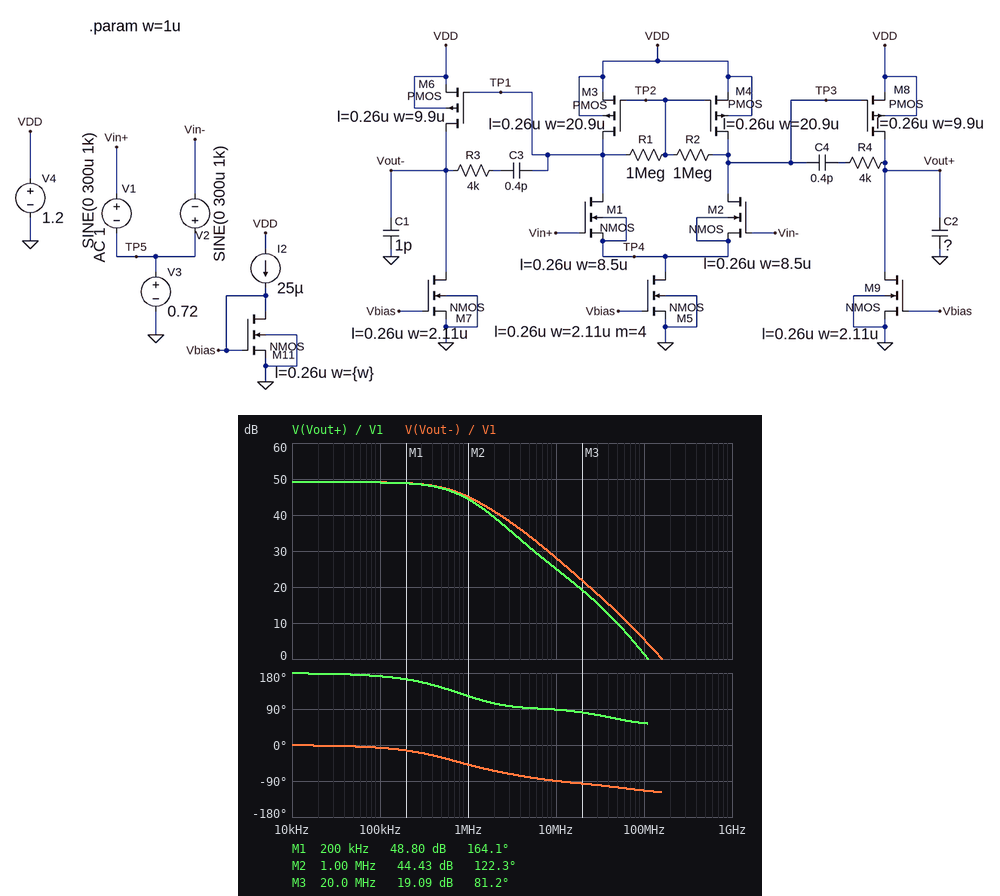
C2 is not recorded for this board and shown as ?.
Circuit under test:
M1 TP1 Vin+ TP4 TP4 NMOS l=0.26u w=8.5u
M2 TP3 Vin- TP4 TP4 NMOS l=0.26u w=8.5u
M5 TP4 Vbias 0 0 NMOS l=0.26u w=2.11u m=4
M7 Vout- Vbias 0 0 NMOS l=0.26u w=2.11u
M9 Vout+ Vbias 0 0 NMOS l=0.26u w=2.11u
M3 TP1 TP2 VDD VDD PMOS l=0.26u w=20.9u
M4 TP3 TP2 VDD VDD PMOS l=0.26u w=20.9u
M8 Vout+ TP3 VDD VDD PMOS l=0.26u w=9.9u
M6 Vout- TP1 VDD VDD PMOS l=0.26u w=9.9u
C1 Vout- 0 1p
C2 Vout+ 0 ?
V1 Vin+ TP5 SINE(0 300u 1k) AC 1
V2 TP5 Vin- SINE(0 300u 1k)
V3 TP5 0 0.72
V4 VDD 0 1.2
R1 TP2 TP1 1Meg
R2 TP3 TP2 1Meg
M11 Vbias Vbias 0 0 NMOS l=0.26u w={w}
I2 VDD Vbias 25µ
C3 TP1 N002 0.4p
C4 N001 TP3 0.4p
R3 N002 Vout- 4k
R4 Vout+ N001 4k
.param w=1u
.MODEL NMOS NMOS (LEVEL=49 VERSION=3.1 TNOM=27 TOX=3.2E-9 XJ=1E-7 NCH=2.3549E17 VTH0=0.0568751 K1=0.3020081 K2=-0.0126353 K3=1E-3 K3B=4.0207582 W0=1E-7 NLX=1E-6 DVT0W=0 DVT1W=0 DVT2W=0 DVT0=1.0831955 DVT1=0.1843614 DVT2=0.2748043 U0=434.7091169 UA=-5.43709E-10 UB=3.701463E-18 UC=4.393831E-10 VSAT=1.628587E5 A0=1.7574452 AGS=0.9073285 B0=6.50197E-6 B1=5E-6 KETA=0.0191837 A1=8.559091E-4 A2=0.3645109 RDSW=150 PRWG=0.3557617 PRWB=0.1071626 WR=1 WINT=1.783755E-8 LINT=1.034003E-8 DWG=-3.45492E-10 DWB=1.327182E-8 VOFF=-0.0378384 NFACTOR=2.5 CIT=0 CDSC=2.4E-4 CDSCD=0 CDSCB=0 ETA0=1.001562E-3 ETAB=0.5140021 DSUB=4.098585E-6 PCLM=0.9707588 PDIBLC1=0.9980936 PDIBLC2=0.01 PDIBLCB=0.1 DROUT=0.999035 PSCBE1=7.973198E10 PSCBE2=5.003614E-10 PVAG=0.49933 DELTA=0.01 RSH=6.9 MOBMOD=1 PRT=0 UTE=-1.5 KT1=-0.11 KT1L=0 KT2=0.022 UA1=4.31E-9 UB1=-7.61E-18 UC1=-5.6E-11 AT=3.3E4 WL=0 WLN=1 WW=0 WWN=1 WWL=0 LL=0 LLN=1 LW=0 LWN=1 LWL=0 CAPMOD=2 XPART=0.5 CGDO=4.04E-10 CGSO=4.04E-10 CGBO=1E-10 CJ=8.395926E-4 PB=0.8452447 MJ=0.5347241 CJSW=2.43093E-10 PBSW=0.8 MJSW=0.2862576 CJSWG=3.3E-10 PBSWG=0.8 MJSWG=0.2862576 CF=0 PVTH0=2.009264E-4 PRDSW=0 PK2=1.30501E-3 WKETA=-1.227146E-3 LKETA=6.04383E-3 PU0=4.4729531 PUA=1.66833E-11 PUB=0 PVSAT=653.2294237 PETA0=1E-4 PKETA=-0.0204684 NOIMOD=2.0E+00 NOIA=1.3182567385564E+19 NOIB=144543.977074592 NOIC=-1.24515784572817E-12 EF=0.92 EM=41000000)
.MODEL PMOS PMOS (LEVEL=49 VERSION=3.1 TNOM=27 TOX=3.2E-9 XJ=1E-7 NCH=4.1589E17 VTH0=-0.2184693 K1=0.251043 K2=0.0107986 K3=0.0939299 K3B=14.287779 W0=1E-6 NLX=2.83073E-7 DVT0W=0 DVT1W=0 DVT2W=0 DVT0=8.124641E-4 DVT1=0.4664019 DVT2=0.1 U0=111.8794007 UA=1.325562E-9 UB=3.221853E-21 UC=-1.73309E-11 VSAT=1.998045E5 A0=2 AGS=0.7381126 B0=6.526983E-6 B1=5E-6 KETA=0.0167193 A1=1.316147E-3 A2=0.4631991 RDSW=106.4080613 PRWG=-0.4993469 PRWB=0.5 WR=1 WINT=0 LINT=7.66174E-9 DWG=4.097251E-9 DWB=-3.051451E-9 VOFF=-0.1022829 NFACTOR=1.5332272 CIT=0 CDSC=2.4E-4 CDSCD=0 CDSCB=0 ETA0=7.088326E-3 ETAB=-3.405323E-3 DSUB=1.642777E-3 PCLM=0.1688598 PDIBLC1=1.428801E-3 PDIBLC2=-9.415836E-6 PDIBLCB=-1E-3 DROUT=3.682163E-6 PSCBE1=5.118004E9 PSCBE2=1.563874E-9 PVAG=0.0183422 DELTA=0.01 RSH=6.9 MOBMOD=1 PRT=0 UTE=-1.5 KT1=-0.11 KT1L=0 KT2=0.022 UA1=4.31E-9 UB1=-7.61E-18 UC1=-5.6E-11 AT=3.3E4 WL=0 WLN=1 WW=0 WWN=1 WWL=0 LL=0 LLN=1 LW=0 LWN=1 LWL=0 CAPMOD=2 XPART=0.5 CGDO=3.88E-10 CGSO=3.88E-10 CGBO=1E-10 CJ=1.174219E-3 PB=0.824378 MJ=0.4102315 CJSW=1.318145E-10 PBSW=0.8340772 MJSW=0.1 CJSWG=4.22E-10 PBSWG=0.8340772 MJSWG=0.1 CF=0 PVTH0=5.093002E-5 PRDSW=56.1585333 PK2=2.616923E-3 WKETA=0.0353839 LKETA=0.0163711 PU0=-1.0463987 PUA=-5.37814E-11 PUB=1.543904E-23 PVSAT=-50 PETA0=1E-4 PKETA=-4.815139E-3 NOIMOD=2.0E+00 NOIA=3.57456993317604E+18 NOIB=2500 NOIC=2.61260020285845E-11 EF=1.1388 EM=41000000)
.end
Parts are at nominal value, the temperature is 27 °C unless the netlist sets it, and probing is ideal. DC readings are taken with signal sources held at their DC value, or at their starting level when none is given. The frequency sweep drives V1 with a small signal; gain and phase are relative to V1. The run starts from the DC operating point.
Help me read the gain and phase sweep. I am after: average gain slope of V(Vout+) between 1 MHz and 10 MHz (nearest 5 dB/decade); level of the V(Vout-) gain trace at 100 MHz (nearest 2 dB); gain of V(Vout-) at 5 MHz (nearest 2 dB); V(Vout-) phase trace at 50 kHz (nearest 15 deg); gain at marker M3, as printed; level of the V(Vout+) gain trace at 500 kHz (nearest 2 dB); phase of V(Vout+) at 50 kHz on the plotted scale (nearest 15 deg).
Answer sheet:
-20 dB/decade
6 dB
34 dB
0 deg
19.09 dB
48 dB
180 deg
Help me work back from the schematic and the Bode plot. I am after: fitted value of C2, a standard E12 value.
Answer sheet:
1.8 pF
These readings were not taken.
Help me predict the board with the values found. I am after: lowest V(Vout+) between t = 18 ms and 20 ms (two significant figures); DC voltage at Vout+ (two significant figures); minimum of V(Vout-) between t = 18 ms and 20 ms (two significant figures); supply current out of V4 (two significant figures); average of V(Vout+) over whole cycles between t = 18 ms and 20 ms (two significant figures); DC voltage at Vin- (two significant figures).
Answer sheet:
230 mV
370 mV
230 mV
330 µA
380 mV
720 mV
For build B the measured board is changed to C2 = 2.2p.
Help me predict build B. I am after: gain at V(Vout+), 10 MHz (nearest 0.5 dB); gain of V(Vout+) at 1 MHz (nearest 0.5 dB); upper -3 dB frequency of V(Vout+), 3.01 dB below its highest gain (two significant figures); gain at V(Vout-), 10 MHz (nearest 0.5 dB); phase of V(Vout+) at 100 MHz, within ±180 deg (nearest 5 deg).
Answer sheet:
24.0 dB
44.0 dB
690 kHz
28.5 dB
50 deg
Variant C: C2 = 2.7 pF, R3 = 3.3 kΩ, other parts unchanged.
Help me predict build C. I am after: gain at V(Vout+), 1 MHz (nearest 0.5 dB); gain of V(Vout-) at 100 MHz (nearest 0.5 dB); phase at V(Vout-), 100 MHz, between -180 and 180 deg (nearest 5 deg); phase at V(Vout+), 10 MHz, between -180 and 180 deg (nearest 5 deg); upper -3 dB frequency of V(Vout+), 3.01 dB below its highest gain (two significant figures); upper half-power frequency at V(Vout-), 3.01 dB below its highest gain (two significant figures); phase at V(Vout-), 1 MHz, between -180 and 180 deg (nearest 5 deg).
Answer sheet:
43.5 dB
5.0 dB
-120 deg
85 deg
650 kHz
780 kHz
-45 deg
